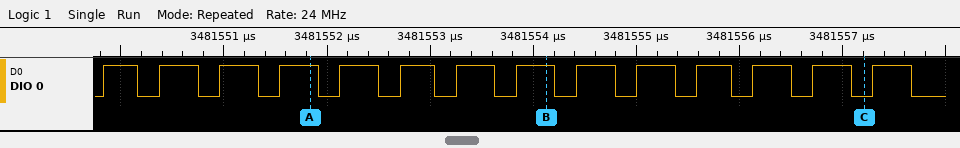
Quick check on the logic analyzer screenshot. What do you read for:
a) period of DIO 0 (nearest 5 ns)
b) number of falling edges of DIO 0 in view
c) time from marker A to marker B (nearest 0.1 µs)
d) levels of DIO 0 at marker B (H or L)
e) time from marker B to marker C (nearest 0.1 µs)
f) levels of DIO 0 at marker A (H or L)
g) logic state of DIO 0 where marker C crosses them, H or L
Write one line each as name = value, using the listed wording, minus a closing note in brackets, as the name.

period of DIO 0 = 575 ns
number of falling edges of DIO 0 in view = 14
time from marker A to marker B = 2.3 µs
levels of DIO 0 at marker B = DIO 0=H
time from marker B to marker C = 3.1 µs
levels of DIO 0 at marker A = DIO 0=H
logic state of DIO 0 where marker C crosses them, H or L = DIO 0=L
